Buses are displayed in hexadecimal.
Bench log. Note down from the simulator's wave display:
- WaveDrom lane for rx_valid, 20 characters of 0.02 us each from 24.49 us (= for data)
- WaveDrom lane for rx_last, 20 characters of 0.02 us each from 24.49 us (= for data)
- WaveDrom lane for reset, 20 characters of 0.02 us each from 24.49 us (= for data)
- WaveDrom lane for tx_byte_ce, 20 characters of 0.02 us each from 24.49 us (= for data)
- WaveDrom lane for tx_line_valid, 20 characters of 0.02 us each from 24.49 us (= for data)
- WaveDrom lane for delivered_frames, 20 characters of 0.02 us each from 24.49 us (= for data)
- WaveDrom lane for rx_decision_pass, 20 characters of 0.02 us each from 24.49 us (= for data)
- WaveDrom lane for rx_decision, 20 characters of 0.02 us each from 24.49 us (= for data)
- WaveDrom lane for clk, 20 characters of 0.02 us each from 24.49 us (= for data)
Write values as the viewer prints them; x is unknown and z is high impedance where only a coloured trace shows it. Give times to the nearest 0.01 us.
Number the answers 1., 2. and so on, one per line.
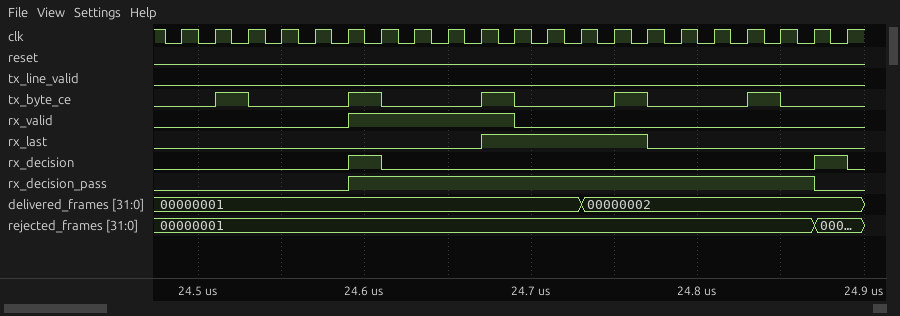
1. {name: 'rx_valid', wave: '0....1....0.........'}
2. {name: 'rx_last', wave: '0........1....0.....'}
3. {name: 'reset', wave: '0...................'}
4. {name: 'tx_byte_ce', wave: '010..10..10..10..10.'}
5. {name: 'tx_line_valid', wave: '0...................'}
6. {name: 'delivered_frames', wave: '=...........=.......', data: '00000001 00000002'}
7. {name: 'rx_decision_pass', wave: '0....1.............0'}
8. {name: 'rx_decision', wave: '0....10............1'}
9. {name: 'clk', wave: 'p...................'}
